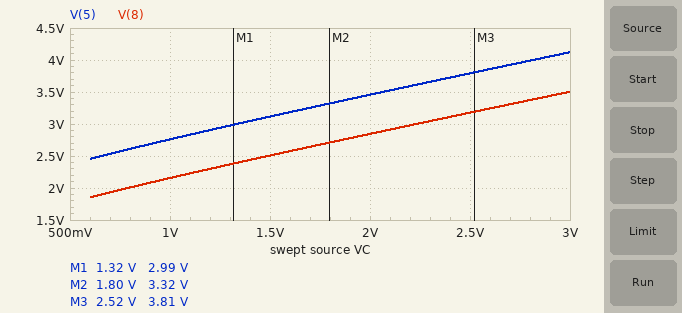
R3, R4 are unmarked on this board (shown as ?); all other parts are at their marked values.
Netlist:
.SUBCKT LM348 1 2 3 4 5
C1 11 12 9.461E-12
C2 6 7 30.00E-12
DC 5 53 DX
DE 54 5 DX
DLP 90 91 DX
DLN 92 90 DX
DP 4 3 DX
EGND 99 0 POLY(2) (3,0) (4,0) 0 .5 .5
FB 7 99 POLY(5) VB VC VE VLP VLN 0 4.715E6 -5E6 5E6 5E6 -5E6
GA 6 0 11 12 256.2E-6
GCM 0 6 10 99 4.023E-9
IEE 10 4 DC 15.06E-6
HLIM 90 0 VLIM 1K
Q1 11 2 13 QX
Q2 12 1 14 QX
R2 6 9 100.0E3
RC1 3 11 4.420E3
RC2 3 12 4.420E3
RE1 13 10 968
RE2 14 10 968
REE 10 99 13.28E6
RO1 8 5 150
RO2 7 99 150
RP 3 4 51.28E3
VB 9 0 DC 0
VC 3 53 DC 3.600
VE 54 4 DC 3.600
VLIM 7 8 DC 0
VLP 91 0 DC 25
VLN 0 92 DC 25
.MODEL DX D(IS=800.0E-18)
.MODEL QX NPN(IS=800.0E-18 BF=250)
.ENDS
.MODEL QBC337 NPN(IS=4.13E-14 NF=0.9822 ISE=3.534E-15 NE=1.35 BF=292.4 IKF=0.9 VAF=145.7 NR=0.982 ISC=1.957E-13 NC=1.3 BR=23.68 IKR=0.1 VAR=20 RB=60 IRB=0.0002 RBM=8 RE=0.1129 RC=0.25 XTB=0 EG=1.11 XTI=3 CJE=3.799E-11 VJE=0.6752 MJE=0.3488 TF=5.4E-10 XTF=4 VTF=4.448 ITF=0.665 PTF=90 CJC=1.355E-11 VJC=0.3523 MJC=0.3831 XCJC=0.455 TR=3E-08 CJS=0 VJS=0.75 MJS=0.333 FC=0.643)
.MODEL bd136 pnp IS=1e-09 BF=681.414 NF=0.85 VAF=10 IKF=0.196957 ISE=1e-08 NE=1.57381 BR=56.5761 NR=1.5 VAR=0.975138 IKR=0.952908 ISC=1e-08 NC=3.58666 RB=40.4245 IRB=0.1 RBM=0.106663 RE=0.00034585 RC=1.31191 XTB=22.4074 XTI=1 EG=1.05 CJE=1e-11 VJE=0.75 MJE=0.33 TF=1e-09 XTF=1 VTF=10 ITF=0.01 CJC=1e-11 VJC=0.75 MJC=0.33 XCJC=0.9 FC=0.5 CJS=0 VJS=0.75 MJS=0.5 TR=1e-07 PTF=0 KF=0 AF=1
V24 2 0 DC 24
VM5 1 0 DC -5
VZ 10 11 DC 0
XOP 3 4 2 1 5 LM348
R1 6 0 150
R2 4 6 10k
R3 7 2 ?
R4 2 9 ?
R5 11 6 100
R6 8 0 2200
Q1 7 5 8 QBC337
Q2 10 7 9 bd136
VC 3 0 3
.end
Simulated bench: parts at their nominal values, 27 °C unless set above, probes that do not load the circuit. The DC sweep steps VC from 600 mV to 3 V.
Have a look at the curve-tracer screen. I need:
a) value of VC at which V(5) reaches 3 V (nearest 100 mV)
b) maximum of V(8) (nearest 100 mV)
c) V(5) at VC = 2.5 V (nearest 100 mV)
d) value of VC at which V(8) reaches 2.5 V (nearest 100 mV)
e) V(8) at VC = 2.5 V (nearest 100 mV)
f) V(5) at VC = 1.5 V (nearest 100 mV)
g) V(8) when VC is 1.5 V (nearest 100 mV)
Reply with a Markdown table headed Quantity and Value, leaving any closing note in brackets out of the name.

| Quantity | Value |
|---|---|
| value of VC at which V(5) reaches 3 V | 1.3 V |
| maximum of V(8) | 3.5 V |
| V(5) at VC = 2.5 V | 3.8 V |
| value of VC at which V(8) reaches 2.5 V | 1.5 V |
| V(8) at VC = 2.5 V | 3.2 V |
| V(5) at VC = 1.5 V | 3.1 V |
| V(8) when VC is 1.5 V | 2.5 V |
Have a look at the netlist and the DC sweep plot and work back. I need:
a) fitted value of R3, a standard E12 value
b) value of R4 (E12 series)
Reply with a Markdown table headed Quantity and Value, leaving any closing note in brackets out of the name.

| Quantity | Value |
|---|---|
| fitted value of R3, a standard E12 value | 470 Ω |
| value of R4 | 18 Ω |
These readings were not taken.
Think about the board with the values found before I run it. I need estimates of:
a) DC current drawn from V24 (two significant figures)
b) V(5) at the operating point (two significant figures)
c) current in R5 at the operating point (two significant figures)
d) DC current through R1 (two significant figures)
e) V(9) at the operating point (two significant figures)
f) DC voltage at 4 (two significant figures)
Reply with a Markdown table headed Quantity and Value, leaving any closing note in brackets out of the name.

| Quantity | Value |
|---|---|
| DC current drawn from V24 | 22 mA |
| V(5) at the operating point | 4.1 V |
| current in R5 at the operating point | 20 mA |
| DC current through R1 | 20 mA |
| V(9) at the operating point | 24 V |
| DC voltage at 4 | 3.0 V |
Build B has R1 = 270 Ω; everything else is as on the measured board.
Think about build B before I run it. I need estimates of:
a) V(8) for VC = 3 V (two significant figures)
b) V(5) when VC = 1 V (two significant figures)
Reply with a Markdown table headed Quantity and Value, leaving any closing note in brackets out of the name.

| Quantity | Value |
|---|---|
| V(8) for VC = 3 V | 2.6 V |
| V(5) when VC = 1 V | 2.4 V |
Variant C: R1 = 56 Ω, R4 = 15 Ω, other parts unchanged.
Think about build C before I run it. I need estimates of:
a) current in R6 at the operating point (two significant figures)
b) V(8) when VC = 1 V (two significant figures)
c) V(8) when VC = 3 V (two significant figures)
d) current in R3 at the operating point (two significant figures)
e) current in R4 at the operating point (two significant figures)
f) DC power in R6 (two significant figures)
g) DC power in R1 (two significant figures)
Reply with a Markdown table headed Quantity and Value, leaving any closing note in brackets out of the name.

| Quantity | Value |
|---|---|
| current in R6 at the operating point | 2.7 mA |
| V(8) when VC = 1 V | 3.0 V |
| V(8) when VC = 3 V | 5.9 V |
| current in R3 at the operating point | 2.5 mA |
| current in R4 at the operating point | 54 mA |
| DC power in R6 | 16 mW |
| DC power in R1 | 160 mW |
